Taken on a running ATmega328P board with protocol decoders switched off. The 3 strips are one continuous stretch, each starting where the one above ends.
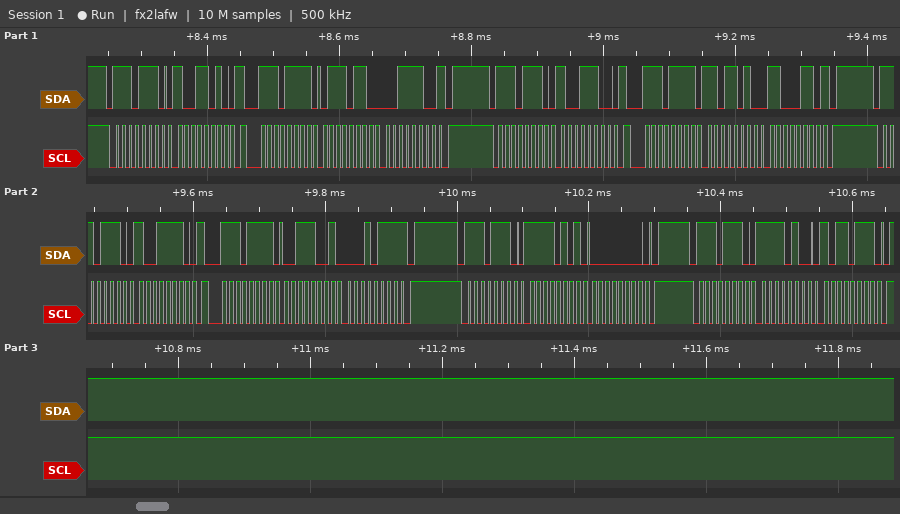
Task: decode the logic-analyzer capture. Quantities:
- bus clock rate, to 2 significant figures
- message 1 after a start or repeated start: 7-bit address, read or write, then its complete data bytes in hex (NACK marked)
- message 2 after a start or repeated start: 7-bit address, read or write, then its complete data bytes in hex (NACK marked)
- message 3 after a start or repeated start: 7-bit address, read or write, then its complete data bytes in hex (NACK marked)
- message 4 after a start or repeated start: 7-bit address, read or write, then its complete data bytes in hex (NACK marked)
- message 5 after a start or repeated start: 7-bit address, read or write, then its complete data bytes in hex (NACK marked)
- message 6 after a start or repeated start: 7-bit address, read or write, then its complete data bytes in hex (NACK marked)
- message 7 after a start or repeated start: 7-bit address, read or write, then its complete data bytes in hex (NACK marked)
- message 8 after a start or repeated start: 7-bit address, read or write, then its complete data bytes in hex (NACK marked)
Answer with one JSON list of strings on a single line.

["100 kHz", "0x77 write: 9A", "0x77 read: 76 3C NACK", "0x77 write: 9C", "0x77 read: DA C6 NACK", "0x77 write: 9E", "0x77 read: 39 17 NACK", "0x77 write: F5 00", "0x77 write: F4 B7"]
